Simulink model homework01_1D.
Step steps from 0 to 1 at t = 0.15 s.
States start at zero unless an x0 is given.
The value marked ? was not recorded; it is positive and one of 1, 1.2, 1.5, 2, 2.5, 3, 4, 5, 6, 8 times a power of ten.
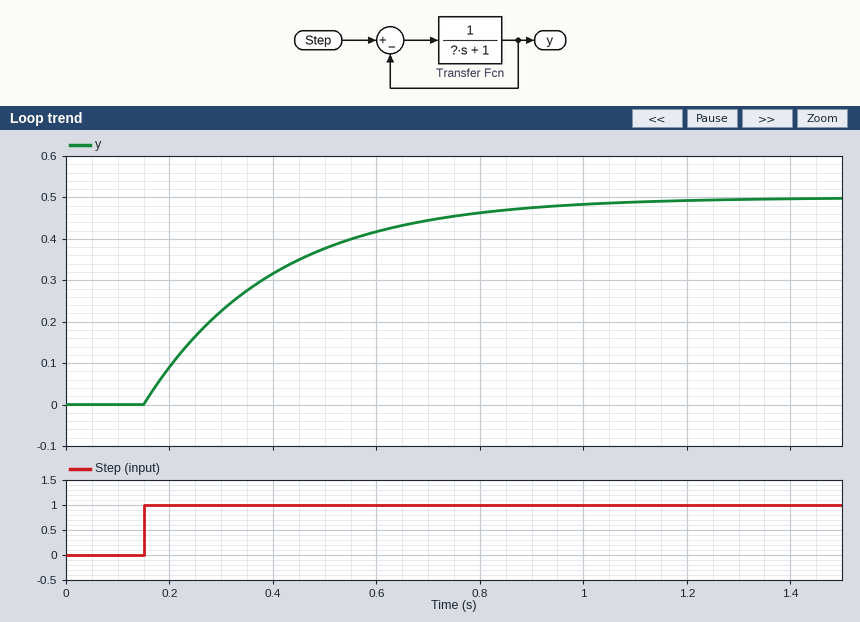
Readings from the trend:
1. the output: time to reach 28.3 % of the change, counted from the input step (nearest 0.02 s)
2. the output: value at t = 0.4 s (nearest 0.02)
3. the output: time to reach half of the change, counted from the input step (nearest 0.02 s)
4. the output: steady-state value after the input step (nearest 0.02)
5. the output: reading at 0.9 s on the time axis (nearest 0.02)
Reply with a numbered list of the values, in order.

1. 0.08 s
2. 0.32
3. 0.18 s
4. 0.50
5. 0.48
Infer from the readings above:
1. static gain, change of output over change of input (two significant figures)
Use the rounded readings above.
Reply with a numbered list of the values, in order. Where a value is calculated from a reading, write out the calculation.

1. (0.5 - 0) / (1 - 0) = 0.50
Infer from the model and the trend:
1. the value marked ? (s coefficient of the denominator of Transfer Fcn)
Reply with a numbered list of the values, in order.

1. 0.5
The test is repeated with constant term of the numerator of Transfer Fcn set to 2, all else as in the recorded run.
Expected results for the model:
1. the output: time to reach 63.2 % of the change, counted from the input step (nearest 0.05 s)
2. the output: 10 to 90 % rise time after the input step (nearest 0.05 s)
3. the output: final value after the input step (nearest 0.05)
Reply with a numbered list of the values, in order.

1. 0.15 s
2. 0.35 s
3. 0.65
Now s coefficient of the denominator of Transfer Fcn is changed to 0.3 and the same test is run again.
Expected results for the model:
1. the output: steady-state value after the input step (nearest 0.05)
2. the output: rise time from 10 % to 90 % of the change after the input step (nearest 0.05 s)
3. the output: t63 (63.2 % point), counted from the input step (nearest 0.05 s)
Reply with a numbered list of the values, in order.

1. 0.50
2. 0.35 s
3. 0.15 s
